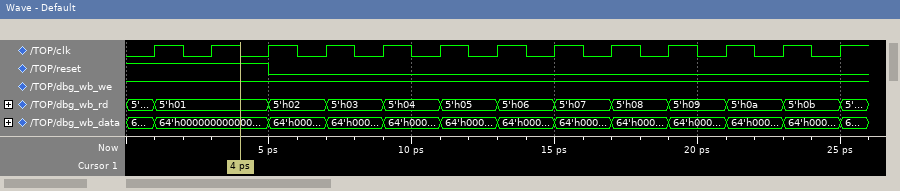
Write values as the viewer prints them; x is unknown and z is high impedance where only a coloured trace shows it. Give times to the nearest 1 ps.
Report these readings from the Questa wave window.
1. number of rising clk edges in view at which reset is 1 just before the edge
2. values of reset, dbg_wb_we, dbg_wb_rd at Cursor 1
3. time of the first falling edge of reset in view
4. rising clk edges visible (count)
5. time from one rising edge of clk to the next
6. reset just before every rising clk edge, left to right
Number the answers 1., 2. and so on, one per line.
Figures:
1. 3
2. reset=1, dbg_wb_we=1, dbg_wb_rd=5'h01
3. 5 ps
4. 13
5. 2 ps
6. 1 1 1 0 0 0 0 0 0 0 0 0 0
